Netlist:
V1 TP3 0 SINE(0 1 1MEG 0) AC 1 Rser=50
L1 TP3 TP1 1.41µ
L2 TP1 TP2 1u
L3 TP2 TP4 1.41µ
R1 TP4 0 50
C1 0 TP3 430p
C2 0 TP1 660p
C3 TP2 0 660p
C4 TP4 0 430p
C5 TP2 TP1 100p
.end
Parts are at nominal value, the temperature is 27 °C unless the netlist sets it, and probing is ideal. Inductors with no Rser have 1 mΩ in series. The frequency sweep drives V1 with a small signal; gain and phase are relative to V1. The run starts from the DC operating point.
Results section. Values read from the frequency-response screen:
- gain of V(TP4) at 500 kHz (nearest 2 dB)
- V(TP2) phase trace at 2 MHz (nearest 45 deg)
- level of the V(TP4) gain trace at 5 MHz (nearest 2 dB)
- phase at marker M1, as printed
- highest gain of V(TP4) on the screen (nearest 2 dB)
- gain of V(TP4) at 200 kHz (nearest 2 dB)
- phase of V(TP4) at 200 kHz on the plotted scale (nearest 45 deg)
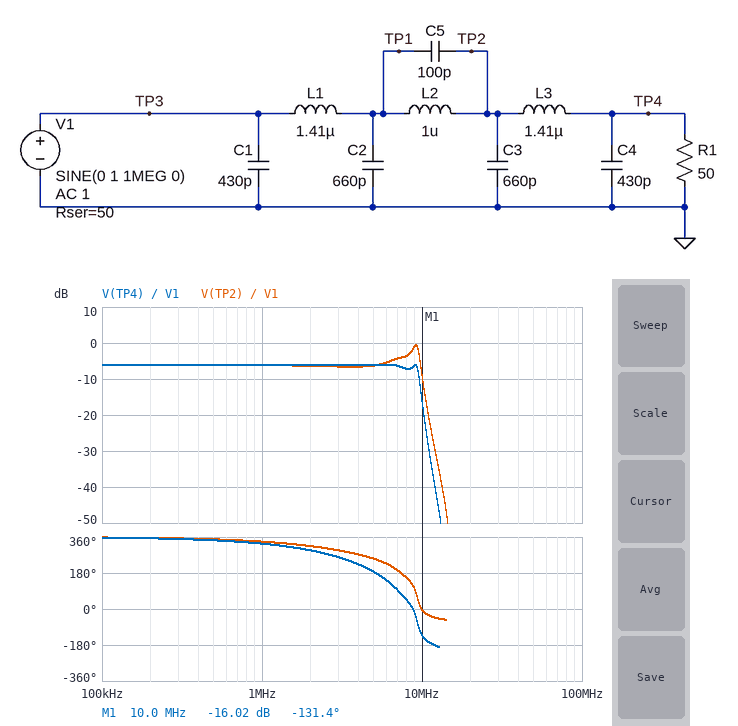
-6 dB
315 deg
-6 dB
-131.4 deg
-6 dB
-6 dB
360 deg
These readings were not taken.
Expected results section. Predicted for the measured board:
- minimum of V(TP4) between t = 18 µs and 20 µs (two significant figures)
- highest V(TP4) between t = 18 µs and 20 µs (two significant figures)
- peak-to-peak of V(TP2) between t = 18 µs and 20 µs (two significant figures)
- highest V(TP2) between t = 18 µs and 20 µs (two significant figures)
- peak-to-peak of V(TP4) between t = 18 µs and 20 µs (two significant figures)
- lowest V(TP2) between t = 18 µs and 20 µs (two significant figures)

-500 mV
500 mV
990 mV
490 mV
1.0 V
-490 mV
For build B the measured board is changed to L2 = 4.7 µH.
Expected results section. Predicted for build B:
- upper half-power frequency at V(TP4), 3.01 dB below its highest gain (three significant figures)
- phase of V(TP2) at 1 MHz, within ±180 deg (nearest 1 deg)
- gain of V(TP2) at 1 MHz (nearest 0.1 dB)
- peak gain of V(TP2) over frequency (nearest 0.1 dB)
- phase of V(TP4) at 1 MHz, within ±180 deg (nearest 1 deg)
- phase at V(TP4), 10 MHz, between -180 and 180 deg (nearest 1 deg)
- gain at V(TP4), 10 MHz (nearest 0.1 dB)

3.03 MHz
-37 deg
-6.2 dB
-6.0 dB
-47 deg
29 deg
-38.0 dB
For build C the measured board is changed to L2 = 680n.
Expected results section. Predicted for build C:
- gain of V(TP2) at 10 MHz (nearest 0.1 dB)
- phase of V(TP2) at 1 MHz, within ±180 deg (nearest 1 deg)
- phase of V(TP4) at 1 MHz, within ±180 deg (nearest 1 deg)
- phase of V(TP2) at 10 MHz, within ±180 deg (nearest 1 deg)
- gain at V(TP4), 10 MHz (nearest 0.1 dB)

-3.4 dB
-22 deg
-32 deg
121 deg
-10.4 dB
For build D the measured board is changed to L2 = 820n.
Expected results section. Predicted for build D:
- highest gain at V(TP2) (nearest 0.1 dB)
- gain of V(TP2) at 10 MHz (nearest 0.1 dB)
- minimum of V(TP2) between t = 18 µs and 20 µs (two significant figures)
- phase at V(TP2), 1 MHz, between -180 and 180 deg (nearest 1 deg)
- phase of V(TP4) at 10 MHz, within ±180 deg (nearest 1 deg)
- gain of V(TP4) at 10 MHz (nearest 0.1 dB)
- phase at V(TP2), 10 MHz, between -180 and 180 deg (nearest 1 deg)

0.8 dB
0.5 dB
-490 mV
-22 deg
-80 deg
-6.6 dB
48 deg
